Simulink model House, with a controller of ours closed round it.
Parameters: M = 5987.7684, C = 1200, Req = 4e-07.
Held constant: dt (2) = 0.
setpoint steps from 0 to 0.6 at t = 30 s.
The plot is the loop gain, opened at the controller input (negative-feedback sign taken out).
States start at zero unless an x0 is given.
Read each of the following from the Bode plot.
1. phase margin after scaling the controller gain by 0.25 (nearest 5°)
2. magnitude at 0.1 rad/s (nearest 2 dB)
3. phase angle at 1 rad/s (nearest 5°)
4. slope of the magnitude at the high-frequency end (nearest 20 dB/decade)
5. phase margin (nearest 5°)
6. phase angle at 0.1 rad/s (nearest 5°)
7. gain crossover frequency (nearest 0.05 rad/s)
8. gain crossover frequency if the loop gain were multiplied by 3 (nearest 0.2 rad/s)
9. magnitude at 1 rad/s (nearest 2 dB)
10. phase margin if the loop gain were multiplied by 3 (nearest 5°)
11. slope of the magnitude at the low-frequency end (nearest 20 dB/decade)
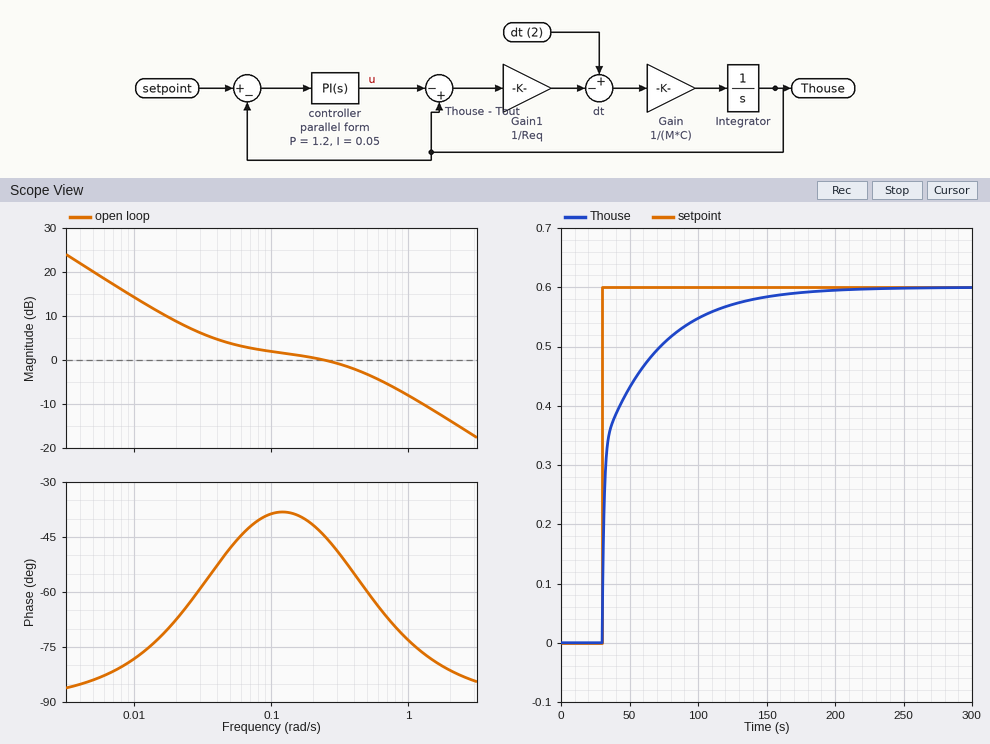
105°
2 dB
-75°
-20 dB/decade
135°
-40°
0.25 rad/s
1.2 rad/s
-8 dB
105°
-20 dB/decade
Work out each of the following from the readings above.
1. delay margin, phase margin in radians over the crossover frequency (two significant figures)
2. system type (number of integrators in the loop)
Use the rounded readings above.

9.4 s
1
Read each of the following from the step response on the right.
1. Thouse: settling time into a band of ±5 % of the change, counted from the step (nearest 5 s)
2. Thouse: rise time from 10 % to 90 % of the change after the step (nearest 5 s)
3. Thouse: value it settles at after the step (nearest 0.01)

95 s
65 s
0.60
